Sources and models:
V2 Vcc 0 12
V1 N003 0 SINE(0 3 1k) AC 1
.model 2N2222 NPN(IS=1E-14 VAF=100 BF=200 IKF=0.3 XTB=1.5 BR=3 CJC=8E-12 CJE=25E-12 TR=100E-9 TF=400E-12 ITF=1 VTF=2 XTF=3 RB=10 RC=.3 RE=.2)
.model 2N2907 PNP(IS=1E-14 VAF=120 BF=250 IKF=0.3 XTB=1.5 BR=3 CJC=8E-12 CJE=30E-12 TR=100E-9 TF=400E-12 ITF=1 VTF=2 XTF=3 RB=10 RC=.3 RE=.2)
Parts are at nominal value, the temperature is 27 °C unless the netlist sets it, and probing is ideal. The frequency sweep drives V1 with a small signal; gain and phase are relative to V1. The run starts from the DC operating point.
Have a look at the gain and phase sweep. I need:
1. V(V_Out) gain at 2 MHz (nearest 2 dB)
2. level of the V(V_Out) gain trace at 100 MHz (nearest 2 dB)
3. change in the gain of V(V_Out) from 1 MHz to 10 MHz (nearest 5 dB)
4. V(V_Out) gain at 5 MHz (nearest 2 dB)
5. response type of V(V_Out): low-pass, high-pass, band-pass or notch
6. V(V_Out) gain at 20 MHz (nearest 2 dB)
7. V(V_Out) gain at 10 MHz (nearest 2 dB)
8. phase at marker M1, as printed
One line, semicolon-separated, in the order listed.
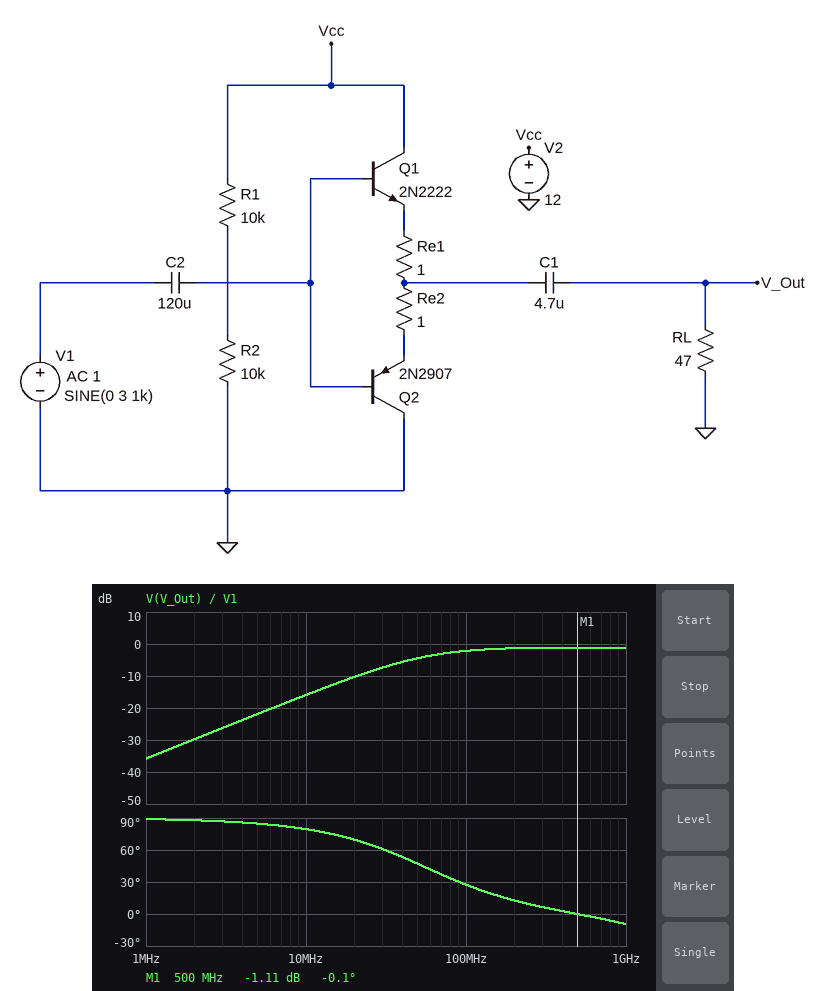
-30 dB; -2 dB; 20 dB; -22 dB; high-pass; -10 dB; -16 dB; -0.1 deg
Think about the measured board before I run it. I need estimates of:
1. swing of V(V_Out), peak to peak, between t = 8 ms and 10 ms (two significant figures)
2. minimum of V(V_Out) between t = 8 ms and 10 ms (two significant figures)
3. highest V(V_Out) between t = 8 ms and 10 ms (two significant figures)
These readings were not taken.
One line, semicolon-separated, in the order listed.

3.8 V; -1.9 V; 1.9 V
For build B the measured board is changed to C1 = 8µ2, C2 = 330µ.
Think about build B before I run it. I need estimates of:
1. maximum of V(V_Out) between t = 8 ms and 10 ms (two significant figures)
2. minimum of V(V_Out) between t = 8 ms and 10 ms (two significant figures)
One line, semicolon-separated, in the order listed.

2.1 V; -2.1 V
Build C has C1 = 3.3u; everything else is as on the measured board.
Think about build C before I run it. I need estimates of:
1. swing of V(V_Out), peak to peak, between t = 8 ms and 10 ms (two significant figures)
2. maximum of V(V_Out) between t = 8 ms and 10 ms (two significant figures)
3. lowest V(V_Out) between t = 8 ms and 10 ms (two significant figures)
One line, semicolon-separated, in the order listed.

3.4 V; 1.7 V; -1.7 V
